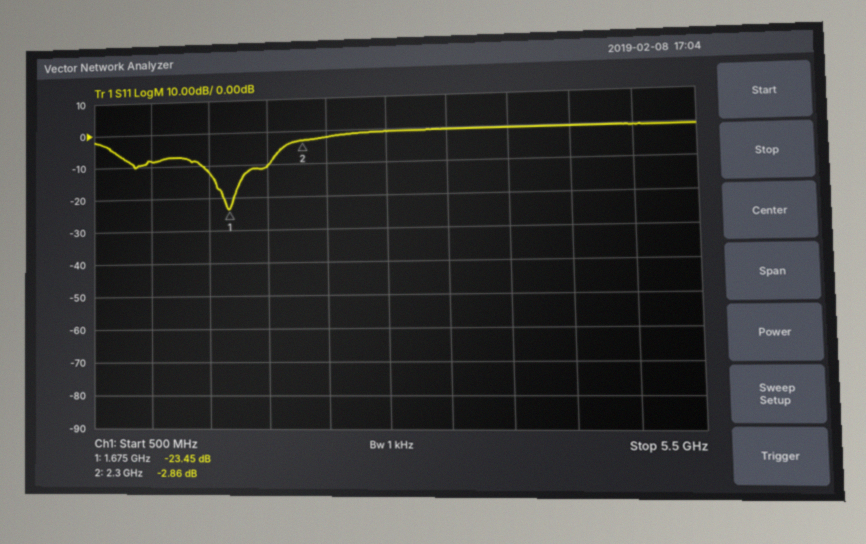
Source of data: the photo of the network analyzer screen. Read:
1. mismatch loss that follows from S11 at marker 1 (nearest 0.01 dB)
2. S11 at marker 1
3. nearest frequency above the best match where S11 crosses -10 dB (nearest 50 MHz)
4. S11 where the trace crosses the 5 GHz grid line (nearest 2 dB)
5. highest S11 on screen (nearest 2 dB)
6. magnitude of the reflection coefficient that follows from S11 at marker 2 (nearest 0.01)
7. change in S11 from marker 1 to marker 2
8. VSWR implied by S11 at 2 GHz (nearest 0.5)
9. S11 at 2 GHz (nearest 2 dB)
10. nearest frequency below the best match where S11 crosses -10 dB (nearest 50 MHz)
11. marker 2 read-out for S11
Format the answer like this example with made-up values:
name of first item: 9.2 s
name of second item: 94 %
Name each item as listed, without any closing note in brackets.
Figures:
mismatch loss that follows from S11 at marker 1: 0.02 dB
S11 at marker 1: -23.45 dB
nearest frequency above the best match where S11 crosses -10 dB: 2.00 GHz
S11 where the trace crosses the 5 GHz grid line: 0 dB
highest S11 on screen: 0 dB
magnitude of the reflection coefficient that follows from S11 at marker 2: 0.72
change in S11 from marker 1 to marker 2: 20.59 dB
VSWR implied by S11 at 2 GHz: 2.0
S11 at 2 GHz: -10 dB
nearest frequency below the best match where S11 crosses -10 dB: 1.45 GHz
marker 2 read-out for S11: -2.86 dB
